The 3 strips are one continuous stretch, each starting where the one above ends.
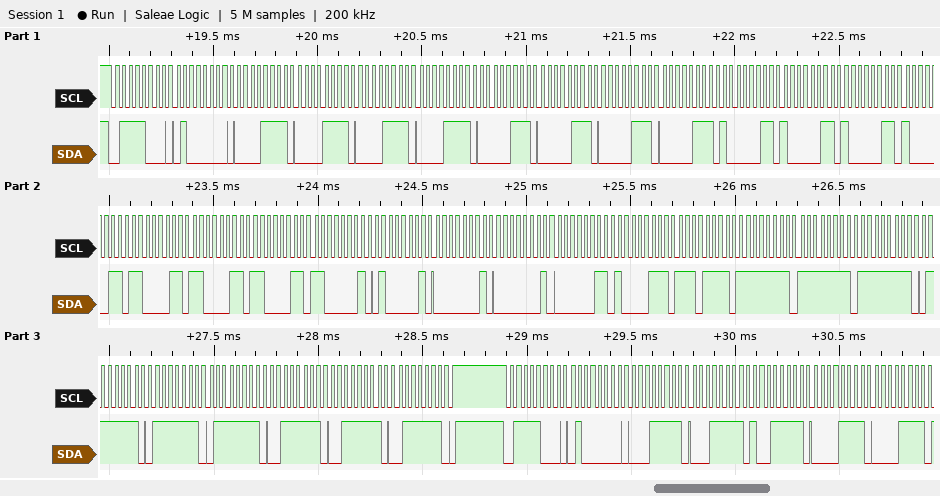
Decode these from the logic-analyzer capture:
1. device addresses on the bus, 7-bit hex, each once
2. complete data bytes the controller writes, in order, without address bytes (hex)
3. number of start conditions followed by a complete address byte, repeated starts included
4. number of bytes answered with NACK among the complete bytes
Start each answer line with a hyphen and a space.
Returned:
- 0x3C
- 40 0F 0F 0F 0F 07 07 07 07 83 83 83 83 C3 C3 C3 C1 41 01 01 03 87 EF FF FF FF 7F 7F 7F 3F 3F 3F 40 1F 1F 9F 0F 0F
- 2
- 0
